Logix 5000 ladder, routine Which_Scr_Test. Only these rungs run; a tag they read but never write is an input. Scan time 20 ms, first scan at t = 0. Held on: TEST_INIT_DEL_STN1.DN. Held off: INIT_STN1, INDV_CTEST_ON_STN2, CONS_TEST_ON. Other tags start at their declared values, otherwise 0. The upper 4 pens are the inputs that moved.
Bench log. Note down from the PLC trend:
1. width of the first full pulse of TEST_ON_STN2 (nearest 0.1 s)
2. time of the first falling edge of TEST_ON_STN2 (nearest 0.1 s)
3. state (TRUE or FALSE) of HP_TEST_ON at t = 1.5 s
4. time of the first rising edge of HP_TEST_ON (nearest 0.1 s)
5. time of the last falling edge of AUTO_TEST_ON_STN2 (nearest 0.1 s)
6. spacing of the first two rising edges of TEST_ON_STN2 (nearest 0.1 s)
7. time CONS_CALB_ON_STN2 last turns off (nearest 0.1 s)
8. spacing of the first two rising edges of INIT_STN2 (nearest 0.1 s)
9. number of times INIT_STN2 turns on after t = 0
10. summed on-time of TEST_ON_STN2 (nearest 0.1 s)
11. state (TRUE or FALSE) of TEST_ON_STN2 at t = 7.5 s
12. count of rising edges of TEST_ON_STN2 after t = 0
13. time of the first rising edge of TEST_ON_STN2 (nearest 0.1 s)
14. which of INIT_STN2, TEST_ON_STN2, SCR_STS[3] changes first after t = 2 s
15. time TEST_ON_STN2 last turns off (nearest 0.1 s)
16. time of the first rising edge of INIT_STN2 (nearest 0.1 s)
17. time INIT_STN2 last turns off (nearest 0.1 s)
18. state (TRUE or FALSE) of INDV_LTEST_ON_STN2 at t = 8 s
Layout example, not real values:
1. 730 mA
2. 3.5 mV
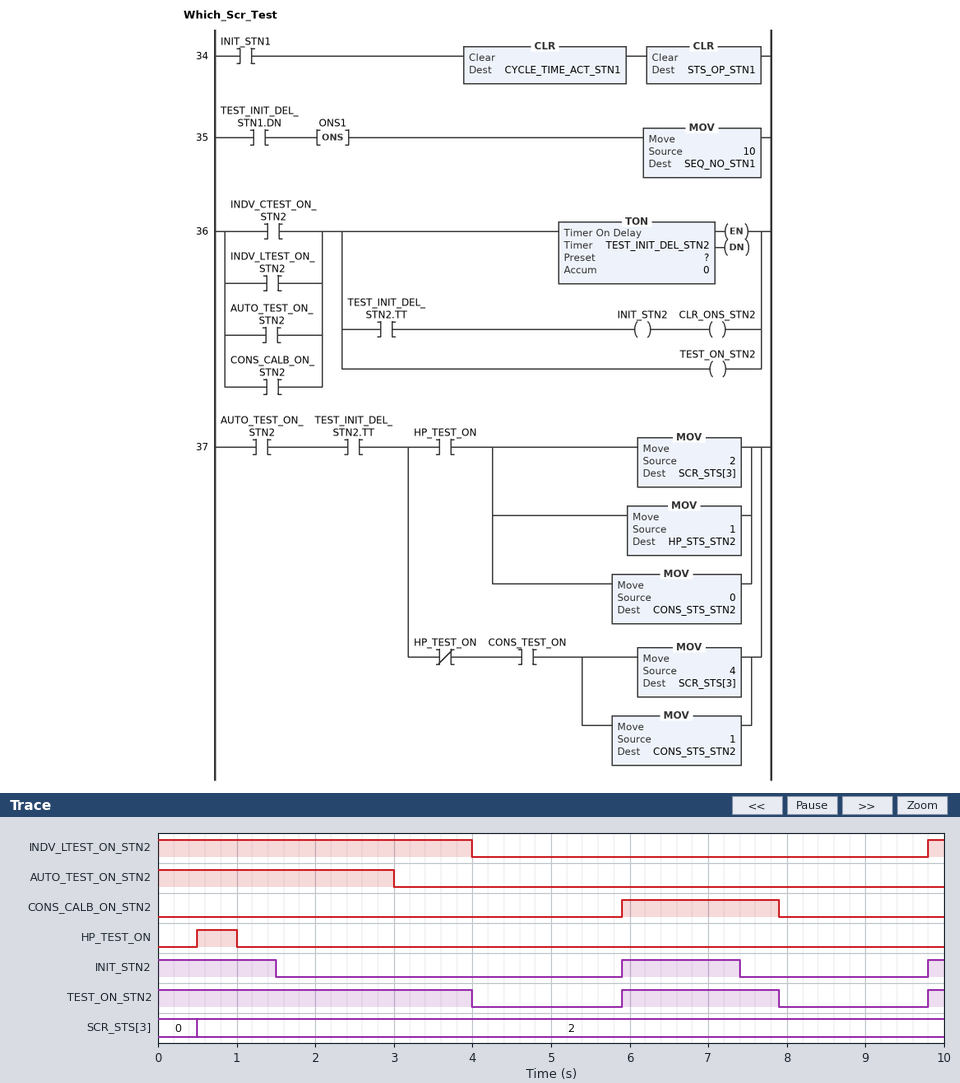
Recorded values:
1. 2.0 s
2. 4.0 s
3. FALSE
4. 0.5 s
5. 3.0 s
6. 3.9 s
7. 7.9 s
8. 3.9 s
9. 2
10. 6.2 s
11. TRUE
12. 2
13. 5.9 s
14. TEST_ON_STN2
15. 7.9 s
16. 5.9 s
17. 7.4 s
18. FALSE
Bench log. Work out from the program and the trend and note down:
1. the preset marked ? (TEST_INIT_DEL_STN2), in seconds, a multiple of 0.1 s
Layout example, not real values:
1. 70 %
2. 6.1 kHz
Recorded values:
1. 1.5 s
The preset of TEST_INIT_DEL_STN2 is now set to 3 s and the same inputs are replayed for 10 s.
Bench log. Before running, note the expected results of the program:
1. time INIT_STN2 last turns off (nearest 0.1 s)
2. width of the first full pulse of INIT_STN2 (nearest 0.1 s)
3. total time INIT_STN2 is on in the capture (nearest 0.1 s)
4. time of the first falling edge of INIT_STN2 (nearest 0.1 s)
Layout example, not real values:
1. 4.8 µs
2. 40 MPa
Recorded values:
1. 7.9 s
2. 2.0 s
3. 5.2 s
4. 3.0 s
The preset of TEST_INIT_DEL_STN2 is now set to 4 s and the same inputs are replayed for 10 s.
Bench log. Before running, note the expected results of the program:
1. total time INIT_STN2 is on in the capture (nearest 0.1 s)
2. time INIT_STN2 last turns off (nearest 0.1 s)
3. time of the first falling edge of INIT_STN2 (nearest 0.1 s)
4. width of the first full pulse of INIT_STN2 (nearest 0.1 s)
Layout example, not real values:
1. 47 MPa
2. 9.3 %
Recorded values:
1. 6.2 s
2. 7.9 s
3. 4.0 s
4. 2.0 s
